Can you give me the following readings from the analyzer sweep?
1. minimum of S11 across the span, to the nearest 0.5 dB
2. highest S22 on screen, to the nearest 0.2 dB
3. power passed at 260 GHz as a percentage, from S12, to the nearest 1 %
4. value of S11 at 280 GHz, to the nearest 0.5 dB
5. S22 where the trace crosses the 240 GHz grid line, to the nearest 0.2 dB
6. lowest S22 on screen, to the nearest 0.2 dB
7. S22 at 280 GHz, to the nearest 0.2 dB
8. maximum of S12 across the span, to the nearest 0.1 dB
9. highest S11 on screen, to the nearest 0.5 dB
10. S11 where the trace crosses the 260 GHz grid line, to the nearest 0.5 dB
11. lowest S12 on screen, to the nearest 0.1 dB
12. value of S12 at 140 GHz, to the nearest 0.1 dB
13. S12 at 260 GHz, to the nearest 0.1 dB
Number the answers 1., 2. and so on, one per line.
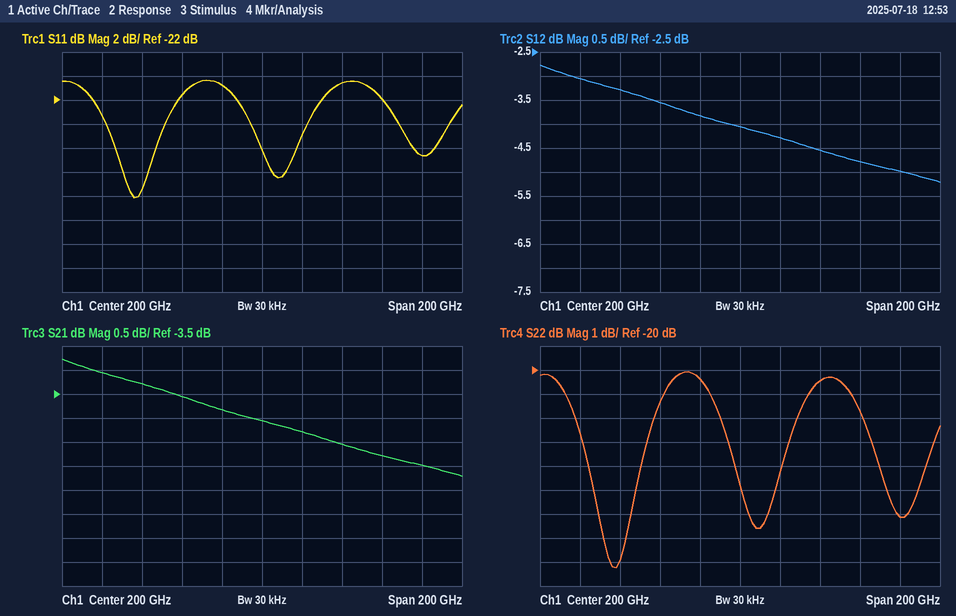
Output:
1. -30.0 dB
2. -20.0 dB
3. 33 %
4. -26.5 dB
5. -20.4 dB
6. -28.2 dB
7. -26.2 dB
8. -2.8 dB
9. -20.5 dB
10. -22.0 dB
11. -5.2 dB
12. -3.3 dB
13. -4.8 dB
